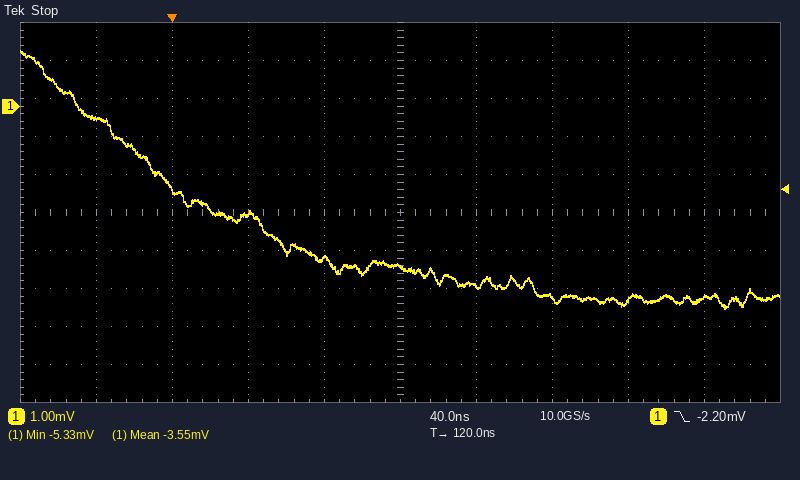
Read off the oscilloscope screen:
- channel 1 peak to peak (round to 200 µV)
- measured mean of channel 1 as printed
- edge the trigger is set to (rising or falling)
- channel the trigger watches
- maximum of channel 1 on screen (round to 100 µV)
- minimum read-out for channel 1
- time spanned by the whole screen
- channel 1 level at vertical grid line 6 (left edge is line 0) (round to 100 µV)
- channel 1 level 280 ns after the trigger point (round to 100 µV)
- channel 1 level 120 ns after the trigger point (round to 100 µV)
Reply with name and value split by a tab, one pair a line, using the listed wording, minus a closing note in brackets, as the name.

channel 1 peak to peak	6.8 mV
measured mean of channel 1 as printed	-3.55 mV
edge the trigger is set to	falling
channel the trigger watches	channel 1
maximum of channel 1 on screen	1.5 mV
minimum read-out for channel 1	-5.33 mV
time spanned by the whole screen	400 ns
channel 1 level at vertical grid line 6 (left edge is line 0)	-4.7 mV
channel 1 level 280 ns after the trigger point	-5.0 mV
channel 1 level 120 ns after the trigger point	-4.2 mV
